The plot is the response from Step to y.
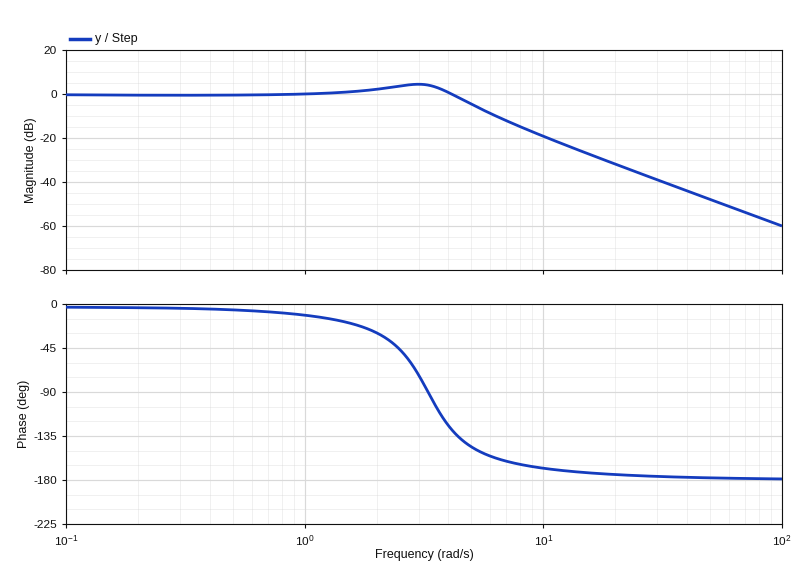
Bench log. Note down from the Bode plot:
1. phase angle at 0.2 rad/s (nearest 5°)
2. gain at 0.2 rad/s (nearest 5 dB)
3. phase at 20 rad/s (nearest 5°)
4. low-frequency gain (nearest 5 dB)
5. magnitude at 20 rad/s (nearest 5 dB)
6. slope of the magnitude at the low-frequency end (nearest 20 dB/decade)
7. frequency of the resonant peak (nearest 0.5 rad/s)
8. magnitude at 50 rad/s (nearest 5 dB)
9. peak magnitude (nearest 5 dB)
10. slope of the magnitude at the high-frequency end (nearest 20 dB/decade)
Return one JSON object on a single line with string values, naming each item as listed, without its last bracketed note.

{"phase angle at 0.2 rad/s": "-5°", "gain at 0.2 rad/s": "0 dB", "phase at 20 rad/s": "-175°", "low-frequency gain": "0 dB", "magnitude at 20 rad/s": "-30 dB", "slope of the magnitude at the low-frequency end": "0 dB/decade", "frequency of the resonant peak": "3.0 rad/s", "magnitude at 50 rad/s": "-50 dB", "peak magnitude": "5 dB", "slope of the magnitude at the high-frequency end": "-40 dB/decade"}
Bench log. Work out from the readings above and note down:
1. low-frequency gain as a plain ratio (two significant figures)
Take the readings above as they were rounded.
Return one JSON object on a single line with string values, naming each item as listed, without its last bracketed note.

{"low-frequency gain as a plain ratio": "1.0"}
